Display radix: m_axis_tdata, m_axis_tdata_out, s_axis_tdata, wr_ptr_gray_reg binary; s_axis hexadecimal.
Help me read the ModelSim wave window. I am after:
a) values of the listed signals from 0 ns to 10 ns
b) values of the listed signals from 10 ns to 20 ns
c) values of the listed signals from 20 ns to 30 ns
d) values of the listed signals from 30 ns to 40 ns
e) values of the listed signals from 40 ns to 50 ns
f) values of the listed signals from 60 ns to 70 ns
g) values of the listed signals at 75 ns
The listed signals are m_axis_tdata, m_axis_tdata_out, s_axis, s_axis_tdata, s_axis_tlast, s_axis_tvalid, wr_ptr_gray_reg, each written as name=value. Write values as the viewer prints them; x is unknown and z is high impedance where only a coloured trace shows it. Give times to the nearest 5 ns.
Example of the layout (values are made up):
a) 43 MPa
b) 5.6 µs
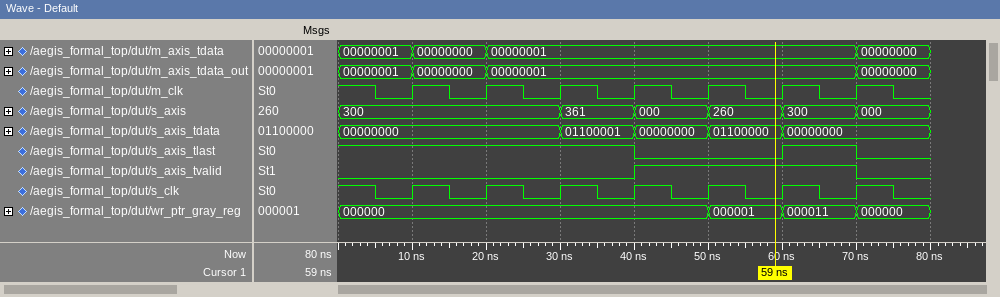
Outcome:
a) m_axis_tdata=00000001, m_axis_tdata_out=00000001, s_axis=300, s_axis_tdata=00000000, s_axis_tlast=1, s_axis_tvalid=0, wr_ptr_gray_reg=000000
b) m_axis_tdata=00000000, m_axis_tdata_out=00000000, s_axis=300, s_axis_tdata=00000000, s_axis_tlast=1, s_axis_tvalid=0, wr_ptr_gray_reg=000000
c) m_axis_tdata=00000001, m_axis_tdata_out=00000001, s_axis=300, s_axis_tdata=00000000, s_axis_tlast=1, s_axis_tvalid=0, wr_ptr_gray_reg=000000
d) m_axis_tdata=00000001, m_axis_tdata_out=00000001, s_axis=361, s_axis_tdata=01100001, s_axis_tlast=1, s_axis_tvalid=0, wr_ptr_gray_reg=000000
e) m_axis_tdata=00000001, m_axis_tdata_out=00000001, s_axis=000, s_axis_tdata=00000000, s_axis_tlast=0, s_axis_tvalid=1, wr_ptr_gray_reg=000000
f) m_axis_tdata=00000001, m_axis_tdata_out=00000001, s_axis=300, s_axis_tdata=00000000, s_axis_tlast=1, s_axis_tvalid=1, wr_ptr_gray_reg=000011
g) m_axis_tdata=00000000, m_axis_tdata_out=00000000, s_axis=000, s_axis_tdata=00000000, s_axis_tlast=0, s_axis_tvalid=0, wr_ptr_gray_reg=000000
